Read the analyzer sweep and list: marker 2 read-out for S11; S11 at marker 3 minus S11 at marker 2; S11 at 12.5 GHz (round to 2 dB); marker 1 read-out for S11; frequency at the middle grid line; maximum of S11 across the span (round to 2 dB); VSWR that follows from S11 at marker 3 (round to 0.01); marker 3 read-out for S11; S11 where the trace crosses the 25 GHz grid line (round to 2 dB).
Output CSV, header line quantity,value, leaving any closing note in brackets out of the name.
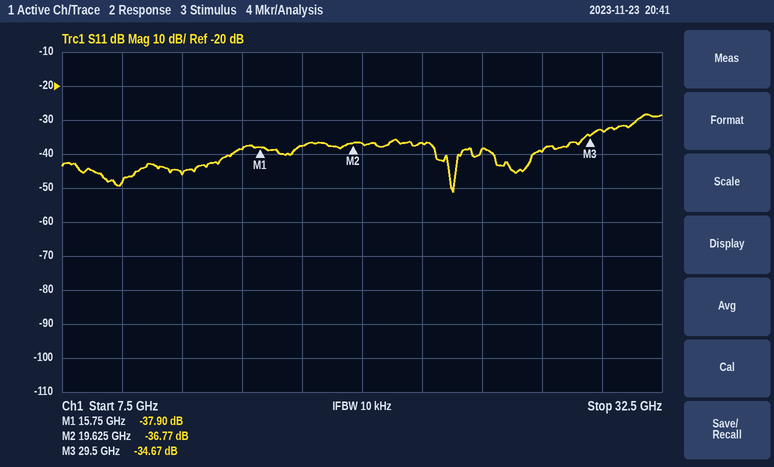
quantity,value
marker 2 read-out for S11,-36.77 dB
S11 at marker 3 minus S11 at marker 2,2.10 dB
S11 at 12.5 GHz,-46 dB
marker 1 read-out for S11,-37.90 dB
frequency at the middle grid line,20 GHz
maximum of S11 across the span,-28 dB
VSWR that follows from S11 at marker 3,1.04
marker 3 read-out for S11,-34.67 dB
S11 where the trace crosses the 25 GHz grid line,-38 dB
